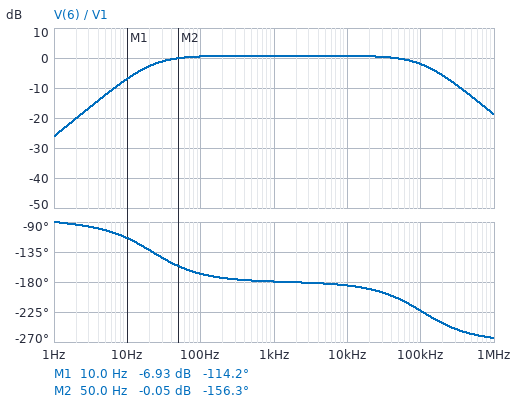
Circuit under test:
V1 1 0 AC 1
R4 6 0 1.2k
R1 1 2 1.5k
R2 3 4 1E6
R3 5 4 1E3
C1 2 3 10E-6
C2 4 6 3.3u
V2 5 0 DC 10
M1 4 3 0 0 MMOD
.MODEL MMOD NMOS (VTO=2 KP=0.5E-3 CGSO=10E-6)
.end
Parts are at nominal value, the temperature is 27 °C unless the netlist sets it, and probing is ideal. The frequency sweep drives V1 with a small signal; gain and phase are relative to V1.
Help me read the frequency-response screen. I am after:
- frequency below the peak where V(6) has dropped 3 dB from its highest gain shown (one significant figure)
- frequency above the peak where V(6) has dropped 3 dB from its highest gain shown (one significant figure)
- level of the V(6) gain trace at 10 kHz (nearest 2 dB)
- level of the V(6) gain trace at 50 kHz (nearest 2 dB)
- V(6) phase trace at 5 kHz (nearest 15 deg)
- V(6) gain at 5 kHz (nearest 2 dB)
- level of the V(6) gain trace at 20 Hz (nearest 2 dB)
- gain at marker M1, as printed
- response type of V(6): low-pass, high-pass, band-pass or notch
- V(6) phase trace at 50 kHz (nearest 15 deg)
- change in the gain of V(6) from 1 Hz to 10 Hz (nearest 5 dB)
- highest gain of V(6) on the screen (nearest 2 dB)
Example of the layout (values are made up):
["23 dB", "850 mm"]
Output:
["20 Hz", "100 kHz", "0 dB", "0 dB", "-180 deg", "0 dB", "-2 dB", "-6.93 dB", "band-pass", "-210 deg", "20 dB", "0 dB"]
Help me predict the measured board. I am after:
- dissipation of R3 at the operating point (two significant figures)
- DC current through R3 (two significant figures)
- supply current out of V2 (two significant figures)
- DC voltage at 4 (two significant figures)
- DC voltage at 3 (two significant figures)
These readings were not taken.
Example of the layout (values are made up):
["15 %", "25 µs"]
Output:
["16 mW", "4.0 mA", "4.0 mA", "6.0 V", "6.0 V"]
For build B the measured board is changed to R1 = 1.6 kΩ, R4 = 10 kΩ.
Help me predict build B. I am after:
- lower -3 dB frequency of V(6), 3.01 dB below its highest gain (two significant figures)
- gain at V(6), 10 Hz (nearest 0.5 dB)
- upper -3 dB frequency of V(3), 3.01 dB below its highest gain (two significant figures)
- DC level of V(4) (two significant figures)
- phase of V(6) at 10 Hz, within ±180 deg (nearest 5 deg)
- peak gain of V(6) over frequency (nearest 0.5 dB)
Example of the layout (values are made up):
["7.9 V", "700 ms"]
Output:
["4.4 Hz", "4.5 dB", "100 kHz", "6.0 V", "-155 deg", "5.0 dB"]
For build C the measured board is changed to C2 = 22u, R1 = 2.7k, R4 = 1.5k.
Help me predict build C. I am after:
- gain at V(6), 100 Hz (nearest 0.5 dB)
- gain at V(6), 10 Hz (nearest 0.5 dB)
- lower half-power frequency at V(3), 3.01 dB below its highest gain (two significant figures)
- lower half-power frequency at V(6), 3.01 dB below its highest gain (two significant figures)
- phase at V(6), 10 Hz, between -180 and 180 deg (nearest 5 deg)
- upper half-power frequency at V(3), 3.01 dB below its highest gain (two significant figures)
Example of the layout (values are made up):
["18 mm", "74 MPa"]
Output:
["1.5 dB", "1.0 dB", "47 mHz", "2.9 Hz", "-165 deg", "59 kHz"]
